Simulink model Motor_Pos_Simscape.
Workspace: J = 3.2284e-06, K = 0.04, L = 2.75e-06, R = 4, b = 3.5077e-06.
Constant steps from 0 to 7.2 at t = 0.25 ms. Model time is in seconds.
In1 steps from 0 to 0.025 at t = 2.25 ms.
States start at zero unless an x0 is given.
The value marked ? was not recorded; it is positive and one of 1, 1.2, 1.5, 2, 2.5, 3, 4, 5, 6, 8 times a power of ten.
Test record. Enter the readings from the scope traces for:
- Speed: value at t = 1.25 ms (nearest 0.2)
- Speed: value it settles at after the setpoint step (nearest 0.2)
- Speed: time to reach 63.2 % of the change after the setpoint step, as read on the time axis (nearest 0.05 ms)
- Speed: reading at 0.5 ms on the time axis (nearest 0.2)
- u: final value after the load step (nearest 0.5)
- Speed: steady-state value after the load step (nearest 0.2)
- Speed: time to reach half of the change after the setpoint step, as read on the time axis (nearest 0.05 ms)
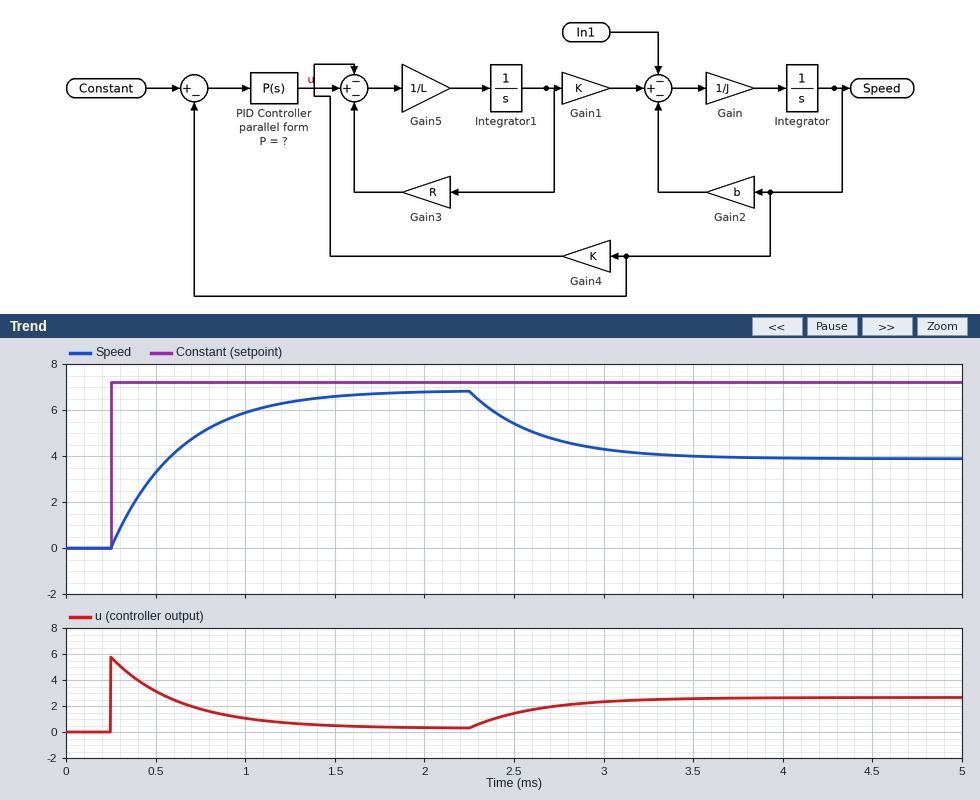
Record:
6.4
6.8
0.65 ms
3.2
2.5
3.8
0.50 ms
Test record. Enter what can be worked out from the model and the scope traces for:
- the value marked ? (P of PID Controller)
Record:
0.8
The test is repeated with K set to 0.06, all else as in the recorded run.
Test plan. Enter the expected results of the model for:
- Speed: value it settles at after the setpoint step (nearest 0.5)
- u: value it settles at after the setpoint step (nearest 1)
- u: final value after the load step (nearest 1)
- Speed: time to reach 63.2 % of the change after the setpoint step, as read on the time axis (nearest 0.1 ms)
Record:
6.5
0
2
0.5 ms
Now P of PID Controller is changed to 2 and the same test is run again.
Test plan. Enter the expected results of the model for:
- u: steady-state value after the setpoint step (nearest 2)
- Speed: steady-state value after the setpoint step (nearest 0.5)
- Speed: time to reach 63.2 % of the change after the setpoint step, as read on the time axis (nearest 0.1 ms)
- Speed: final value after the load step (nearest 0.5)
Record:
0
7.0
0.4 ms
6.0
